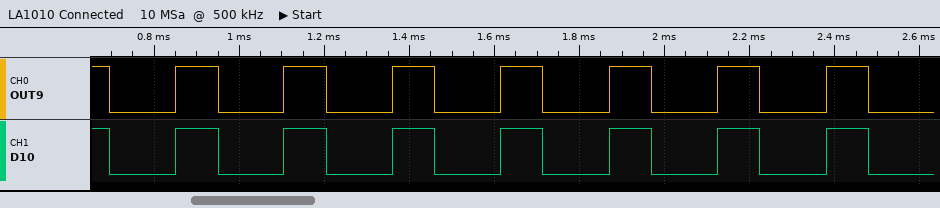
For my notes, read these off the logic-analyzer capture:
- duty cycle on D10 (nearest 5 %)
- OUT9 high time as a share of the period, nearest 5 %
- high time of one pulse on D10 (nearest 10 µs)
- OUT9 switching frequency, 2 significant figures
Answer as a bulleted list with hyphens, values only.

- 40 %
- 40 %
- 100 µs
- 3.9 kHz
